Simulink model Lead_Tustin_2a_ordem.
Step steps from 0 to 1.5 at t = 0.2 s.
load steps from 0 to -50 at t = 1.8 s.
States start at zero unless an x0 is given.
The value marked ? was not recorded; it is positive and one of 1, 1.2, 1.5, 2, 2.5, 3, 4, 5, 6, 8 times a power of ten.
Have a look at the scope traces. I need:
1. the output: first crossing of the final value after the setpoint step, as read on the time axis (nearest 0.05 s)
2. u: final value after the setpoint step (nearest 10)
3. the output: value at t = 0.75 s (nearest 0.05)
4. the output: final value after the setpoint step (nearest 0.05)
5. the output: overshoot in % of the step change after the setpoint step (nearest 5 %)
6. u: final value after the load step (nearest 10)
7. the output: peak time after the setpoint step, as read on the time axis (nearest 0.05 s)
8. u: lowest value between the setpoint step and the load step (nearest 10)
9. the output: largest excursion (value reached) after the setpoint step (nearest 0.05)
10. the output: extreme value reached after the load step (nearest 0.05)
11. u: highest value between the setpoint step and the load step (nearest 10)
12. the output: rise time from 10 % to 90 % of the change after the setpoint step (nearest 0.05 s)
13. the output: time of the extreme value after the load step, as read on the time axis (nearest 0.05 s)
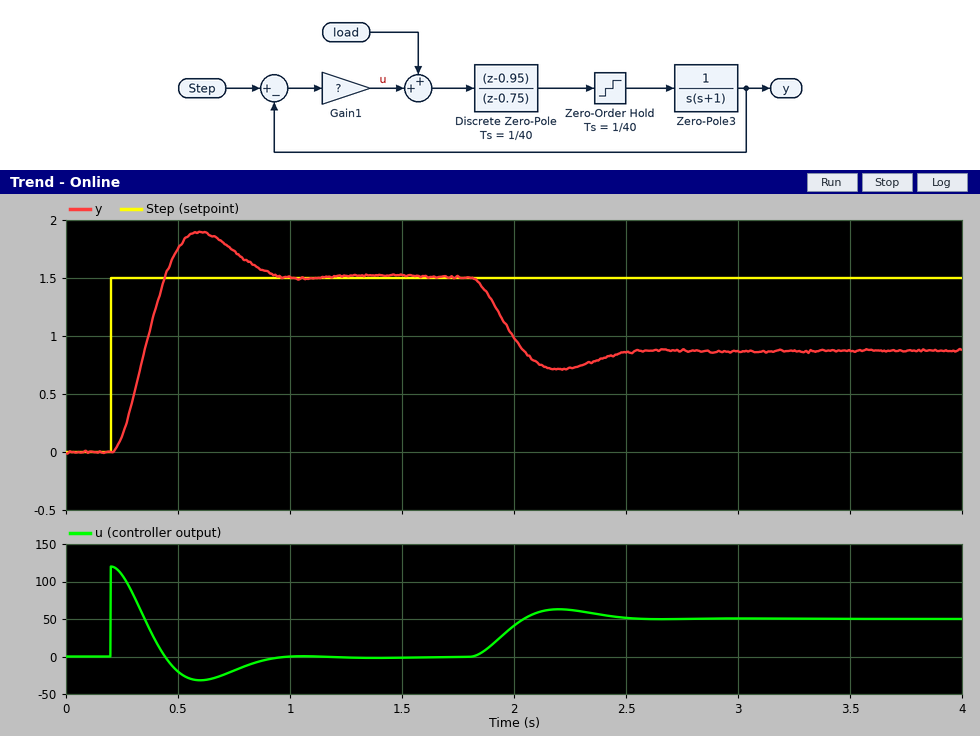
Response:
0.45 s
0
1.75
1.50
25 %
50
0.60 s
-30
1.90
0.70
120
0.15 s
2.20 s
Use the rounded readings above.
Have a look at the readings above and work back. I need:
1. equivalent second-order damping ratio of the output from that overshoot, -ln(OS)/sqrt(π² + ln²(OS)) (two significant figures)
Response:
0.40
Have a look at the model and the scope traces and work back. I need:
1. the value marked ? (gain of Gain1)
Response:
80
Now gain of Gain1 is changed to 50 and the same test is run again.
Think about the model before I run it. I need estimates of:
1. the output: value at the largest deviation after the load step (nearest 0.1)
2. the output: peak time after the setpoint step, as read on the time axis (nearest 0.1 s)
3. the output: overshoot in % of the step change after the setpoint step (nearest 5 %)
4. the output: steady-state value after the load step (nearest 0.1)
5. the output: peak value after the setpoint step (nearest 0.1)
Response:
0.3
0.8 s
20 %
0.5
1.8
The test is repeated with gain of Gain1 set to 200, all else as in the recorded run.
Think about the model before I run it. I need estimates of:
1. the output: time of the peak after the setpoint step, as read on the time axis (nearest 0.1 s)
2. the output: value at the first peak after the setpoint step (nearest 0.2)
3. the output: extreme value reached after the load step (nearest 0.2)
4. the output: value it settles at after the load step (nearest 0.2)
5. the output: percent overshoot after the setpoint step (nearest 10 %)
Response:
0.4 s
2.2
1.2
1.2
50 %
